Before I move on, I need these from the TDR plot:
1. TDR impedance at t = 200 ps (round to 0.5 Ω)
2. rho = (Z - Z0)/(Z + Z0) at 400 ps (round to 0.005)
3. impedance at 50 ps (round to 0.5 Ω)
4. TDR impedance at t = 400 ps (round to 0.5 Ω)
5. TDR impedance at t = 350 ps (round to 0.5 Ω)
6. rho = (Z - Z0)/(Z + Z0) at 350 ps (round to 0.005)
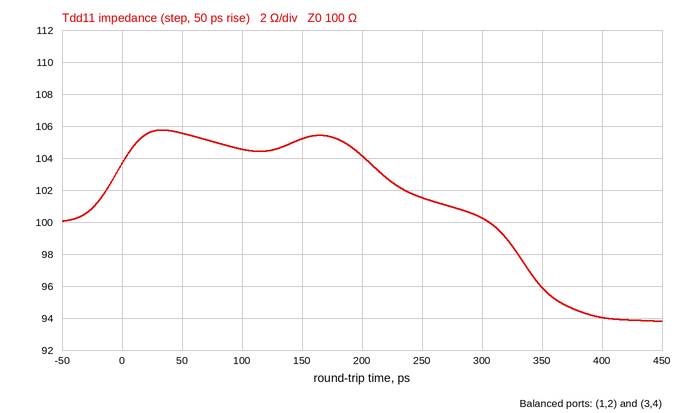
104.0 Ω
-0.030
105.5 Ω
94.0 Ω
96.0 Ω
-0.020
